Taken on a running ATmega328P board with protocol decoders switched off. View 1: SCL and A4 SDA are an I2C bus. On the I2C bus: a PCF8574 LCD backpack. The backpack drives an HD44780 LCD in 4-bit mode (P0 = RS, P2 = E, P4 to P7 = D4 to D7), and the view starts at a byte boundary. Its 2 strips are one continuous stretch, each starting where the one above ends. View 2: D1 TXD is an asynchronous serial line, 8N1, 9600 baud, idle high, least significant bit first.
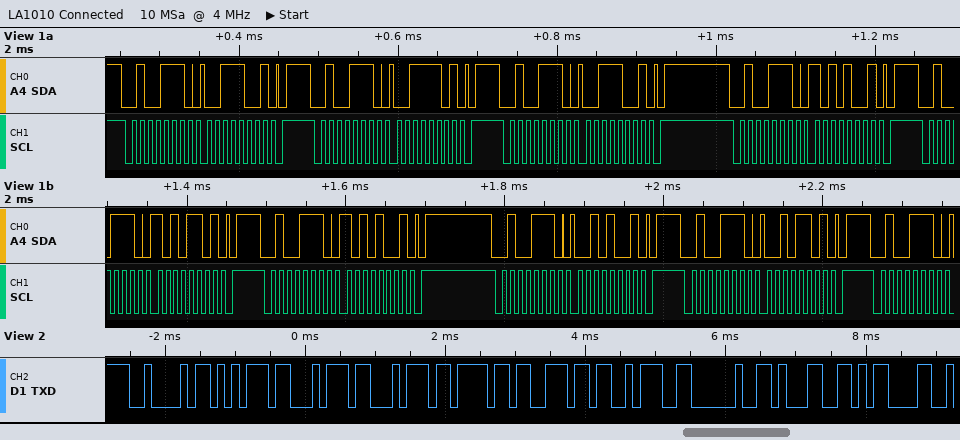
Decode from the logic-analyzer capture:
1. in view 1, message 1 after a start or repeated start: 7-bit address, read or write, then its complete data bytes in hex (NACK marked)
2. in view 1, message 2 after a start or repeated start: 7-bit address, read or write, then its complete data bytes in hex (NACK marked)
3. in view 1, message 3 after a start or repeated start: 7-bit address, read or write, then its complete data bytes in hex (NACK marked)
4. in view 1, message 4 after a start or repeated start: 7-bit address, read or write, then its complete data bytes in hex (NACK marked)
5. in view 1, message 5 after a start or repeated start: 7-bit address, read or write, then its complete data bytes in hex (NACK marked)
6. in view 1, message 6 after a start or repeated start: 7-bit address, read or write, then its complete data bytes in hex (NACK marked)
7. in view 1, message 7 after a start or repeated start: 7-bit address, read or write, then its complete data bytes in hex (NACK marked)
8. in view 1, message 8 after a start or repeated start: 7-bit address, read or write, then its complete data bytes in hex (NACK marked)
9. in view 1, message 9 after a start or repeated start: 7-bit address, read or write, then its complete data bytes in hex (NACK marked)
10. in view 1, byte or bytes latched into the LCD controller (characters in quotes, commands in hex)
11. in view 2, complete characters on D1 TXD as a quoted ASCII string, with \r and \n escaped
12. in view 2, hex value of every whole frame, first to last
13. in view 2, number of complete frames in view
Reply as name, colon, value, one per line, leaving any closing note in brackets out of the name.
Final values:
in view 1, message 1 after a start or repeated start: 7-bit address, read or write, then its complete data bytes in hex: 0x27 write: 39
in view 1, message 2 after a start or repeated start: 7-bit address, read or write, then its complete data bytes in hex: 0x27 write: 3D
in view 1, message 3 after a start or repeated start: 7-bit address, read or write, then its complete data bytes in hex: 0x27 write: 39
in view 1, message 4 after a start or repeated start: 7-bit address, read or write, then its complete data bytes in hex: 0x27 write: A9
in view 1, message 5 after a start or repeated start: 7-bit address, read or write, then its complete data bytes in hex: 0x27 write: AD
in view 1, message 6 after a start or repeated start: 7-bit address, read or write, then its complete data bytes in hex: 0x27 write: A9
in view 1, message 7 after a start or repeated start: 7-bit address, read or write, then its complete data bytes in hex: 0x27 write: 29
in view 1, message 8 after a start or repeated start: 7-bit address, read or write, then its complete data bytes in hex: 0x27 write: 2D
in view 1, message 9 after a start or repeated start: 7-bit address, read or write, then its complete data bytes in hex: 0x27 write
in view 1, byte or bytes latched into the LCD controller: ':'
in view 2, complete characters on D1 TXD as a quoted ASCII string, with \r and \n escaped: "Button: 1\r"
in view 2, hex value of every whole frame, first to last: 42 75 74 74 6F 6E 3A 20 31 0D
in view 2, number of complete frames in view: 10
